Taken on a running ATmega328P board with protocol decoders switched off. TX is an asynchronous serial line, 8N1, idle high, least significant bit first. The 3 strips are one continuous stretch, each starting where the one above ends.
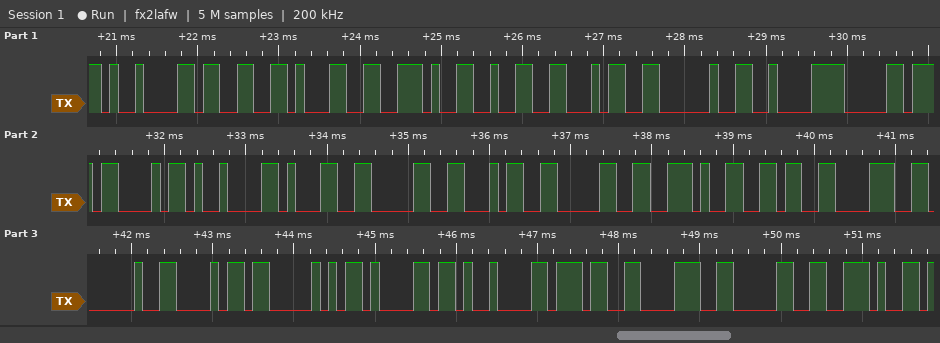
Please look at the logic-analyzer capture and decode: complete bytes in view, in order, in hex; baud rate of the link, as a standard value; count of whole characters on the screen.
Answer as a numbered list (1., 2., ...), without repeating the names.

1. 09 33 31 2E 32 34 20 C2 B0 43 09 31 30 34 30 2E 36 38 20 68 50 61 09 37 38 30 2E
2. 9600 baud
3. 27
